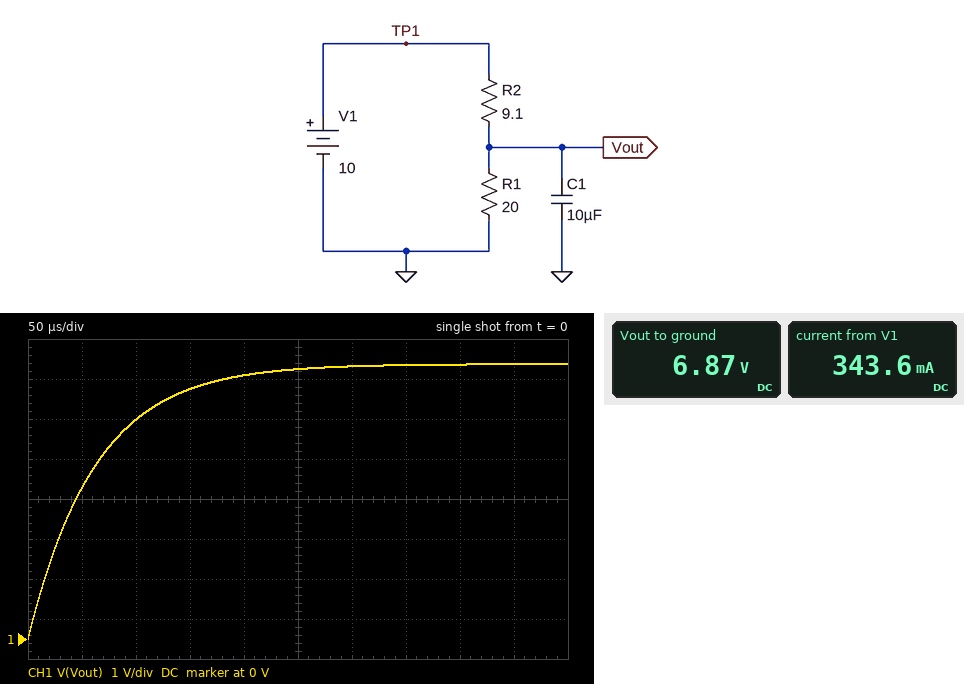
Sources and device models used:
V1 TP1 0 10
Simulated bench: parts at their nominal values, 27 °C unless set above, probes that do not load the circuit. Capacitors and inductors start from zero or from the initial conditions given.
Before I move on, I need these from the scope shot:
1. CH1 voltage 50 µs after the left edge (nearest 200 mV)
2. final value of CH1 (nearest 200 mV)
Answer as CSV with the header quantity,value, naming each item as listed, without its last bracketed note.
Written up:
quantity,value
CH1 voltage 50 µs after the left edge,3.8 V
final value of CH1,6.8 V
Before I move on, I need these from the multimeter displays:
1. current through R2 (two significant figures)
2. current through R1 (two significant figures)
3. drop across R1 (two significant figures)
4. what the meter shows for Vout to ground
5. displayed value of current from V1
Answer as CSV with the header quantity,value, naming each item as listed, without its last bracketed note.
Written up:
quantity,value
current through R2,340 mA
current through R1,340 mA
drop across R1,6.9 V
what the meter shows for Vout to ground,6.87 V
displayed value of current from V1,343.6 mA
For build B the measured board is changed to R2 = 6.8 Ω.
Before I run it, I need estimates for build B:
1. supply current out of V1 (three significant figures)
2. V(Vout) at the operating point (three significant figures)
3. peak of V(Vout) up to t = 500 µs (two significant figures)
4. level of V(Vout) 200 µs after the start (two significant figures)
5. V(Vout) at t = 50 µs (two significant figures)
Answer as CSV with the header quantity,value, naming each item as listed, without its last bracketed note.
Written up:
quantity,value
supply current out of V1,373 mA
V(Vout) at the operating point,7.46 V
peak of V(Vout) up to t = 500 µs,7.5 V
level of V(Vout) 200 µs after the start,7.3 V
V(Vout) at t = 50 µs,4.7 V
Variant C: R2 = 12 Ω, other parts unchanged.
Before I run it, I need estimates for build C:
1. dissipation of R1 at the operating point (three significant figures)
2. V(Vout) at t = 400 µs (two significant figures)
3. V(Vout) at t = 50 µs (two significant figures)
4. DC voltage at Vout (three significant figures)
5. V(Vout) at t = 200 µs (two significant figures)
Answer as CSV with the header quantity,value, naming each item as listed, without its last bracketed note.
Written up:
quantity,value
dissipation of R1 at the operating point,1.95 W
V(Vout) at t = 400 µs,6.2 V
V(Vout) at t = 50 µs,3.0 V
DC voltage at Vout,6.25 V
V(Vout) at t = 200 µs,5.8 V
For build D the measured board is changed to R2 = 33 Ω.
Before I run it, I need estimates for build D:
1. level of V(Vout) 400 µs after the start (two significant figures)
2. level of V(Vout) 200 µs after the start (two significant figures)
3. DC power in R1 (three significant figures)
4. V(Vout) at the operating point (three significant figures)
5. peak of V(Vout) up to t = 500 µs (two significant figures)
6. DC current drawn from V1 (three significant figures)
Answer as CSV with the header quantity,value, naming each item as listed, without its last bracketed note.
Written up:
quantity,value
level of V(Vout) 400 µs after the start,3.6 V
level of V(Vout) 200 µs after the start,3.0 V
DC power in R1,712 mW
V(Vout) at the operating point,3.77 V
peak of V(Vout) up to t = 500 µs,3.7 V
DC current drawn from V1,189 mA
